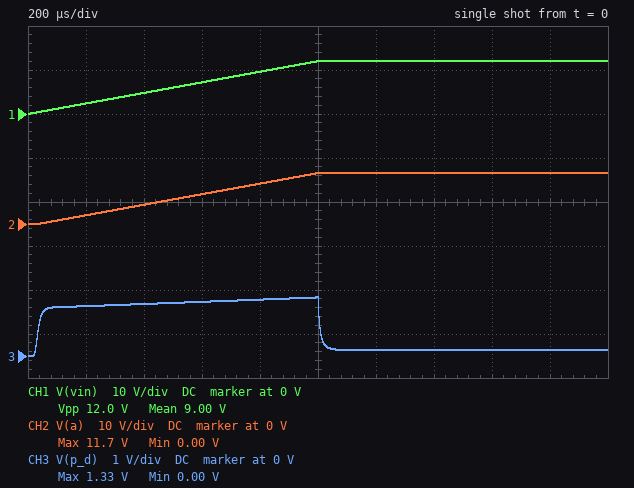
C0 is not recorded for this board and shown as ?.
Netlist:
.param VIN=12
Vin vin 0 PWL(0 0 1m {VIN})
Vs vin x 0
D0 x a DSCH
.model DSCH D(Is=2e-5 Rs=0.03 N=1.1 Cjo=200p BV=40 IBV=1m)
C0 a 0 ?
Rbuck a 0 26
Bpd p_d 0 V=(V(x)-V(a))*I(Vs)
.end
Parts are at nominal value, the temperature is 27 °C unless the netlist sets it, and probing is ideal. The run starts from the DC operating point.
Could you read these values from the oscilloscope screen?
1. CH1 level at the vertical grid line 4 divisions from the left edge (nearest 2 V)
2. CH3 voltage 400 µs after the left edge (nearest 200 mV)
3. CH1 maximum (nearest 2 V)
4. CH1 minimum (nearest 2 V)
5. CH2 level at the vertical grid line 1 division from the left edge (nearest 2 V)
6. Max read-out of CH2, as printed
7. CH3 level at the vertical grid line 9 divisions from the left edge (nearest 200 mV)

10 V
1.2 V
12 V
0 V
2 V
11.7 V
200 mV
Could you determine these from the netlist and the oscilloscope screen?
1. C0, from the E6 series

220 µF
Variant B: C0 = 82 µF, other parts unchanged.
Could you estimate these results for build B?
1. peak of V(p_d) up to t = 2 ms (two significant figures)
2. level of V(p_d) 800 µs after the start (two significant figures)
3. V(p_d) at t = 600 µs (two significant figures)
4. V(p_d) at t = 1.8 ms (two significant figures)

520 mV
480 mV
440 mV
130 mV
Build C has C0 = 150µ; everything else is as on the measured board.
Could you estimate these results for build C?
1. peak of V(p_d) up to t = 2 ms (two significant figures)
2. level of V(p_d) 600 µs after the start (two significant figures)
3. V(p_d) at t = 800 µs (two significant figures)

890 mV
800 mV
850 mV
